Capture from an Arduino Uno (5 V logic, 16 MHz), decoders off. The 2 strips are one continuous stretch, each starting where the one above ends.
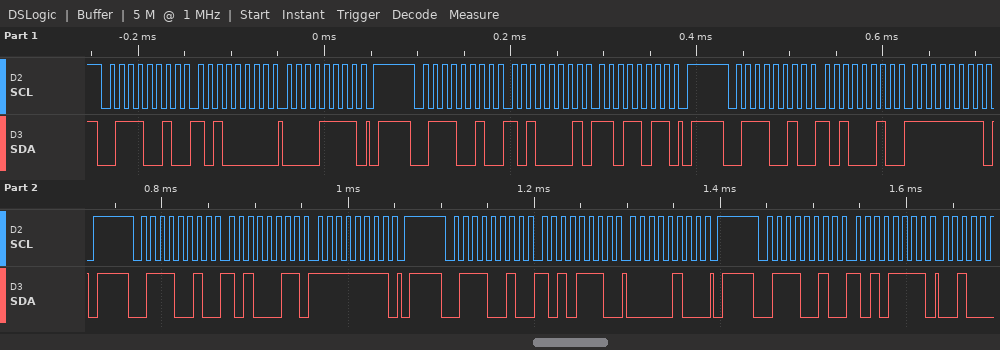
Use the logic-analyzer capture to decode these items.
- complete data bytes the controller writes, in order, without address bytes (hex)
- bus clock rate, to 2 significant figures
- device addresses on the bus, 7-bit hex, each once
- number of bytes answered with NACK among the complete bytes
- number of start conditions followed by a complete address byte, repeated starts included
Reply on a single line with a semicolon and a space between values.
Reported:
A0 0F A1 DB A2 FF A3 FF AE 04 AF; 100 kHz; 0x39; 0; 6
